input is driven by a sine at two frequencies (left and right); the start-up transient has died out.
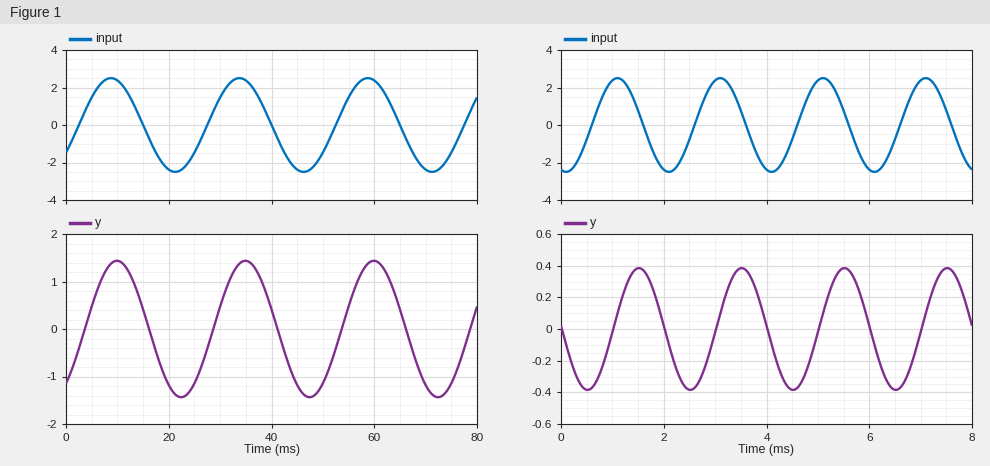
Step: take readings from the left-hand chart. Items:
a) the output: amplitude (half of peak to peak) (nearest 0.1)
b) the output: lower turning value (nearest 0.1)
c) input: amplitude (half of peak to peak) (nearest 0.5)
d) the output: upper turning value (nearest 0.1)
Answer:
1.4
-1.4
2.5
1.4
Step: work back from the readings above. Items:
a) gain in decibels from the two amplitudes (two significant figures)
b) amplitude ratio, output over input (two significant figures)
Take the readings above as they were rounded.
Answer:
-5.0 dB
0.56
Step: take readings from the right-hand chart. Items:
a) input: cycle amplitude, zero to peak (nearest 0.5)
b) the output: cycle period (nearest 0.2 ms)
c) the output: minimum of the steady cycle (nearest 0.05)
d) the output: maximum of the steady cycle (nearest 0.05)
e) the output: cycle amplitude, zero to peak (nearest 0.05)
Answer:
2.5
2.0 ms
-0.40
0.40
0.40
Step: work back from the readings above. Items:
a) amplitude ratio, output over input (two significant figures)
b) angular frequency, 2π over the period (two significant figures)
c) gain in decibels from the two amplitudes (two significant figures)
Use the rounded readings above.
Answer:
0.16
3.1 rad/ms
-16 dB
